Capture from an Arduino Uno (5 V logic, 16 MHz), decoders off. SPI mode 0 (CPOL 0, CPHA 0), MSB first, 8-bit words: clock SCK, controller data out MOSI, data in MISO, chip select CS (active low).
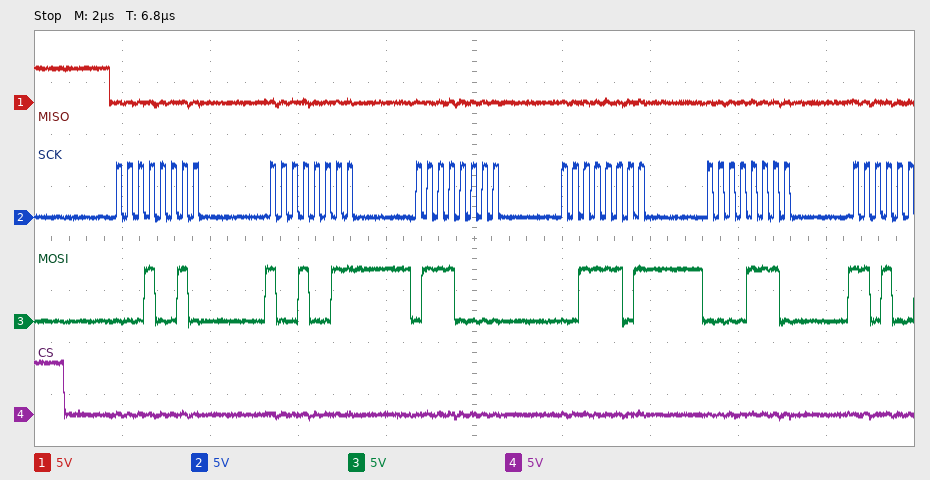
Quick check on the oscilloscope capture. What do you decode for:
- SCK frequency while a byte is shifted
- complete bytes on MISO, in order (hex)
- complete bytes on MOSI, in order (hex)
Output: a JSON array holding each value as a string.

["4 MHz", "00 00 00 00 00", "12 93 70 3D 0E"]
